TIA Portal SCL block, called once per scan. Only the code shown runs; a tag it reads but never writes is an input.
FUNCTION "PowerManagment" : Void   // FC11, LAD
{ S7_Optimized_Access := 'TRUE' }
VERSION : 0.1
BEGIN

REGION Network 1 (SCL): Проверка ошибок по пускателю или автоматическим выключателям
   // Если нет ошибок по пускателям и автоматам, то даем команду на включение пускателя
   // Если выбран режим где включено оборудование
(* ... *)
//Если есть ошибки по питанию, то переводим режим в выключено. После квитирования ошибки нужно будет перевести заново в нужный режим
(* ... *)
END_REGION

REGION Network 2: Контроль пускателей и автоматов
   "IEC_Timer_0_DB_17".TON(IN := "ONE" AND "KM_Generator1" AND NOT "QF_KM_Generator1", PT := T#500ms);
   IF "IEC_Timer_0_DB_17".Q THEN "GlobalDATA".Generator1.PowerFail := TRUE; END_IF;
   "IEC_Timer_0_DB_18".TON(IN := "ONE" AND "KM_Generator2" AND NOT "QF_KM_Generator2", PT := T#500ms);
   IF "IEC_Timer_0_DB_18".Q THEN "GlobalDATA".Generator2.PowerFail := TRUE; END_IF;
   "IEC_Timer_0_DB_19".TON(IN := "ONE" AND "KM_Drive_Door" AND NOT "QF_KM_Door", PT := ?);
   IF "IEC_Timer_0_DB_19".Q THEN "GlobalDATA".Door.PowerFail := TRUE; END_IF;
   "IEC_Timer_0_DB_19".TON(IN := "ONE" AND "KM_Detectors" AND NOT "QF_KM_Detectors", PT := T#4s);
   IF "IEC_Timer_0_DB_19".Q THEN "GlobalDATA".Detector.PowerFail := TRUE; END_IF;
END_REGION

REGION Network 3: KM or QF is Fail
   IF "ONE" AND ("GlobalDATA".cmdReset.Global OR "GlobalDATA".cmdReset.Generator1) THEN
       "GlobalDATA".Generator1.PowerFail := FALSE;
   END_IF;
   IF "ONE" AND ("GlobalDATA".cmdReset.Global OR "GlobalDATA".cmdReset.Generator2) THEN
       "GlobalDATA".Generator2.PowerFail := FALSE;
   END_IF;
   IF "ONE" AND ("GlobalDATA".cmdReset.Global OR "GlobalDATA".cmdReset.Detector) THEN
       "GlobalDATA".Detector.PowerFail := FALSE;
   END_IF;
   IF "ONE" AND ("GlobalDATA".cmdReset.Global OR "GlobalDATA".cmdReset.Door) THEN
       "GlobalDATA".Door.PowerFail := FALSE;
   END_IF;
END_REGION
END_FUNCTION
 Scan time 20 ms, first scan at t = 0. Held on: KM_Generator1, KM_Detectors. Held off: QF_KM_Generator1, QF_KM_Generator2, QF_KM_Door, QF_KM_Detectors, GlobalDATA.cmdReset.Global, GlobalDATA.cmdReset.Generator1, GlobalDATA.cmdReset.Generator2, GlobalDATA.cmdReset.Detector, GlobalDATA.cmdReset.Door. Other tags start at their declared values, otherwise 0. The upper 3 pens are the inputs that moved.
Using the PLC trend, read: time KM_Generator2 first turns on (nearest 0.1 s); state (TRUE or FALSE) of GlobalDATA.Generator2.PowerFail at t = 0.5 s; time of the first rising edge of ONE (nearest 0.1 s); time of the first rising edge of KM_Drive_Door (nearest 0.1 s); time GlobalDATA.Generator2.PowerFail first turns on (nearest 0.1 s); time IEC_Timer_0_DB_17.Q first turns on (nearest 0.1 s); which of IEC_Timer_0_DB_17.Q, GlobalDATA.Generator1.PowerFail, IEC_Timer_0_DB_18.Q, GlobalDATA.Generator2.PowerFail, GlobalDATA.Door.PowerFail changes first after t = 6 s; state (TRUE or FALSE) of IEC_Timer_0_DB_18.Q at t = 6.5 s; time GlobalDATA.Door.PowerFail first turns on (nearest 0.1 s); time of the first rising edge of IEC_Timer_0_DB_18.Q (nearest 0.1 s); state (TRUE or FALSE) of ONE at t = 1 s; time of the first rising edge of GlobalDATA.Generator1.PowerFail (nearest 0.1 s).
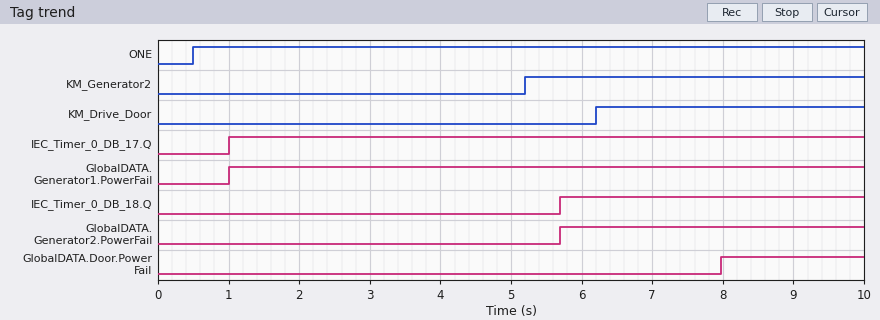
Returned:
5.2 s
FALSE
0.5 s
6.2 s
5.7 s
1.0 s
GlobalDATA.Door.PowerFail
TRUE
8.0 s
5.7 s
TRUE
1.0 s
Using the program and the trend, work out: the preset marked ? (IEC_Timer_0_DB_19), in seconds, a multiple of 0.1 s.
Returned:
1.8 s
